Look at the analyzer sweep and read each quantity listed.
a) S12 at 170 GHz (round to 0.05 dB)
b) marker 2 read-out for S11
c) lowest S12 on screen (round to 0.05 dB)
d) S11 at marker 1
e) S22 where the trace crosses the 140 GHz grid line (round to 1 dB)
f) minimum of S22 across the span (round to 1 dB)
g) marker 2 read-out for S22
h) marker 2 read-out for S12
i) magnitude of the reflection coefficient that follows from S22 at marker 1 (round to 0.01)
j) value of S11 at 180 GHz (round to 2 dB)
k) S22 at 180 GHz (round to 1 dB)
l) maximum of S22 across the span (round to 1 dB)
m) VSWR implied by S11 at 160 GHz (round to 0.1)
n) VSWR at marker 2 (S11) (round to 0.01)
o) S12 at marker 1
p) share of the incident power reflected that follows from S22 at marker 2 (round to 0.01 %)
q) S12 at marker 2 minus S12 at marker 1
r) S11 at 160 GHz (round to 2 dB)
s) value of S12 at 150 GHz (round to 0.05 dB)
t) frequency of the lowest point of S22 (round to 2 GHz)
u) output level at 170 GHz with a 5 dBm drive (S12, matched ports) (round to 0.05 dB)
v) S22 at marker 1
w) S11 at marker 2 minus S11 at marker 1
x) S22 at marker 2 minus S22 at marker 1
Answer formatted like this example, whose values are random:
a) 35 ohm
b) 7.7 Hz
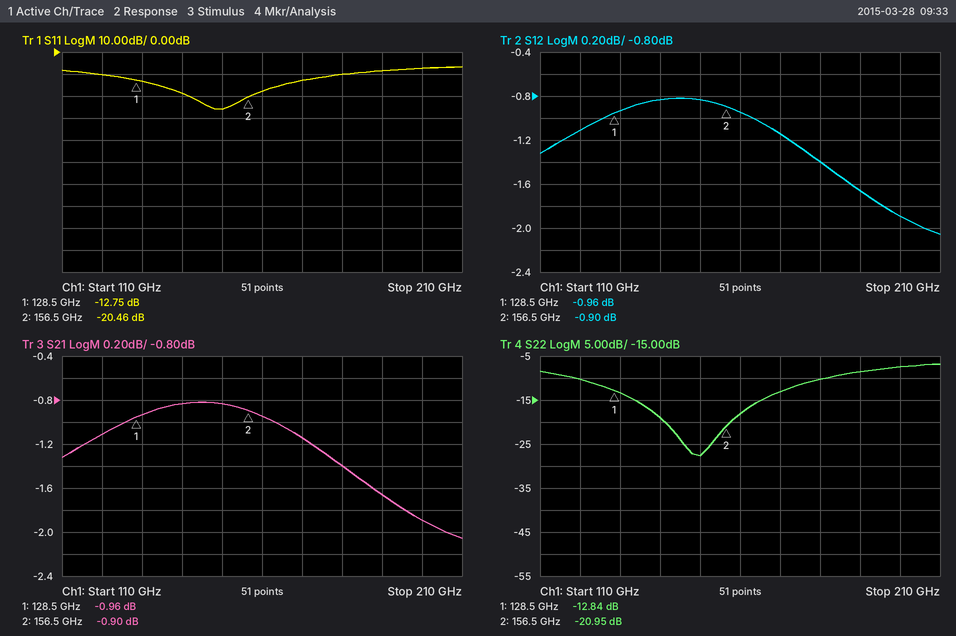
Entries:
a) -1.15 dB
b) -20.46 dB
c) -2.05 dB
d) -12.75 dB
e) -19 dB
f) -28 dB
g) -20.95 dB
h) -0.90 dB
i) 0.23
j) -10 dB
k) -10 dB
l) -7 dB
m) 1.3
n) 1.21
o) -0.96 dB
p) 0.80 %
q) 0.06 dB
r) -18 dB
s) -0.85 dB
t) 150 GHz
u) 3.85 dBm
v) -12.84 dB
w) -7.71 dB
x) -8.11 dB
